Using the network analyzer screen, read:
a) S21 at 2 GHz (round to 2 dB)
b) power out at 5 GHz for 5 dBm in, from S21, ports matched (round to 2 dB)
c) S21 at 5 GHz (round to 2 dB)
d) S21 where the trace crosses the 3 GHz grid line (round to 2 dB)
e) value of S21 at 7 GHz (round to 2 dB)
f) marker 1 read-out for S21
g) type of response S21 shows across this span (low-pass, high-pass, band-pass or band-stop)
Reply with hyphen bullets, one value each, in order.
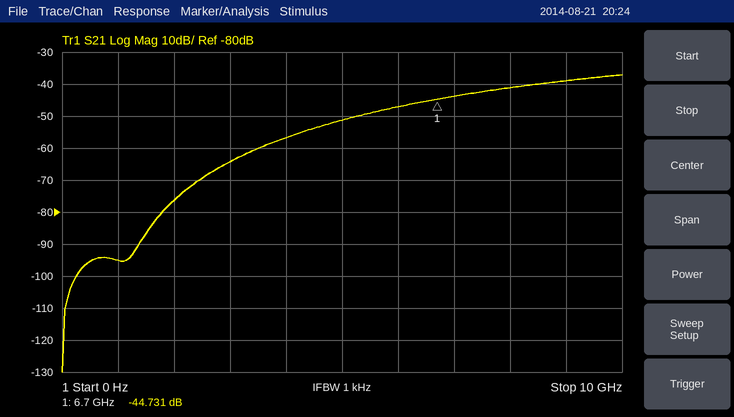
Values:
- -76 dB
- -46 dBm
- -52 dB
- -64 dB
- -44 dB
- -44.731 dB
- high-pass
